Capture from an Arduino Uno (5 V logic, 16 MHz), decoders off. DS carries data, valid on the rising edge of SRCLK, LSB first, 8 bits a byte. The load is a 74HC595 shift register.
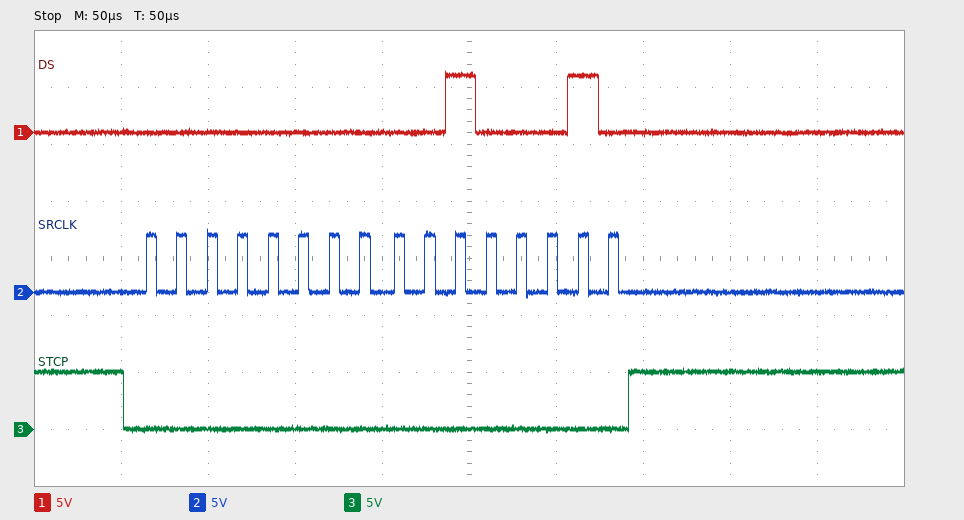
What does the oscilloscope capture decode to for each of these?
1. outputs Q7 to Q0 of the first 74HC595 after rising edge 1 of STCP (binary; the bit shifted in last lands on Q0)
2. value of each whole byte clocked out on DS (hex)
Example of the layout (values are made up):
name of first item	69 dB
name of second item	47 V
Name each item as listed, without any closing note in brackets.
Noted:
outputs Q7 to Q0 of the first 74HC595 after rising edge 1 of STCP	00100010
value of each whole byte clocked out on DS	00 44
